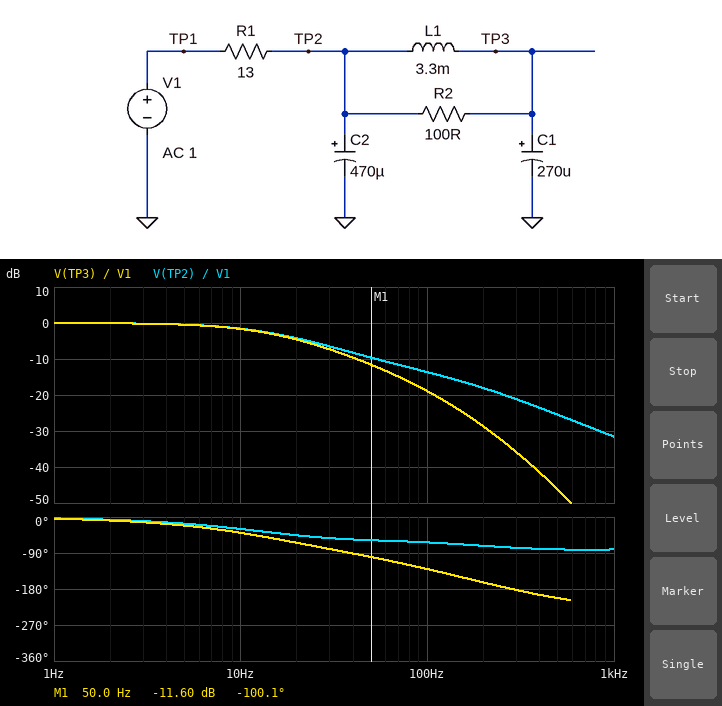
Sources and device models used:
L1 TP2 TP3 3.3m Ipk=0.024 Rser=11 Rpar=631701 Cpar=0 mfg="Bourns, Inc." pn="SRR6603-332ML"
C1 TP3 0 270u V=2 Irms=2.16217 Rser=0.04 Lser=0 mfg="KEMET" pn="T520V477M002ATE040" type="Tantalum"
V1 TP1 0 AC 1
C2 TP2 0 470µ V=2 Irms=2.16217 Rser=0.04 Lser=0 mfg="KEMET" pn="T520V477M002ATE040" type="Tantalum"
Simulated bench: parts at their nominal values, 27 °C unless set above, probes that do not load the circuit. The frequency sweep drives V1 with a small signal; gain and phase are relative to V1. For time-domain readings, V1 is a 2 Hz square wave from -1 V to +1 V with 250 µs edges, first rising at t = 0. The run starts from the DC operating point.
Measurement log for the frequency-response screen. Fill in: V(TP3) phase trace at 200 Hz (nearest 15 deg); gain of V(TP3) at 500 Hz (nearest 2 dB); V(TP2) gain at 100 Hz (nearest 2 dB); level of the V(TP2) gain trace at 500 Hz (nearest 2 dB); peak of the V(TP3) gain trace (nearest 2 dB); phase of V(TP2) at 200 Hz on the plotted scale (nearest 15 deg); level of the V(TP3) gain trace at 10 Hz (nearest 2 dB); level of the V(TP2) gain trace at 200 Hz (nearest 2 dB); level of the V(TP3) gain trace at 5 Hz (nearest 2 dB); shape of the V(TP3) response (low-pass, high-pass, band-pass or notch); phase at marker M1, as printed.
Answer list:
-165 deg
-46 dB
-14 dB
-26 dB
0 dB
-75 deg
-2 dB
-18 dB
0 dB
low-pass
-100.1 deg
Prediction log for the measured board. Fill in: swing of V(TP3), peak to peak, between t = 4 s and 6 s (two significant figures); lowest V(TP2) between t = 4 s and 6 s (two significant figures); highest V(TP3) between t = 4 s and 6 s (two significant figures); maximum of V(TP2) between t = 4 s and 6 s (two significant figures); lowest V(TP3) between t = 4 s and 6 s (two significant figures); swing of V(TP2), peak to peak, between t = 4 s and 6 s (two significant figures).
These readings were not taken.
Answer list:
2.0 V
-1.0 V
1.0 V
1.0 V
-1.0 V
2.0 V
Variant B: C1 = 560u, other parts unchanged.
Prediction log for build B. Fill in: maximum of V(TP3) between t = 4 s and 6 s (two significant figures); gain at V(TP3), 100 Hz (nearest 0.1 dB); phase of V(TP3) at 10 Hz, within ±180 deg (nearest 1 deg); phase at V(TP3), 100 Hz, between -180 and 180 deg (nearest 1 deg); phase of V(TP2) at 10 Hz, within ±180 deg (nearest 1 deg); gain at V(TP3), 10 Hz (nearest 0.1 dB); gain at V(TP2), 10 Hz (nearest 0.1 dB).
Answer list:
1.0 V
-24.3 dB
-54 deg
-142 deg
-35 deg
-3.3 dB
-2.9 dB
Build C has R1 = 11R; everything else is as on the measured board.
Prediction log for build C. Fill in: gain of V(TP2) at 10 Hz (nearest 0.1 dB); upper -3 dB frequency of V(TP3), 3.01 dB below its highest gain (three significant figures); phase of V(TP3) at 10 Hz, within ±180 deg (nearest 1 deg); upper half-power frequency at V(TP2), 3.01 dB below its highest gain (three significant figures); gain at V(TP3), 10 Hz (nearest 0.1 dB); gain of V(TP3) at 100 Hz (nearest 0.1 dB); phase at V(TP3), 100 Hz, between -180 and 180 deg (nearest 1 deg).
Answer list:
-1.2 dB
16.8 Hz
-36 deg
18.0 Hz
-1.3 dB
-17.6 dB
-128 deg
